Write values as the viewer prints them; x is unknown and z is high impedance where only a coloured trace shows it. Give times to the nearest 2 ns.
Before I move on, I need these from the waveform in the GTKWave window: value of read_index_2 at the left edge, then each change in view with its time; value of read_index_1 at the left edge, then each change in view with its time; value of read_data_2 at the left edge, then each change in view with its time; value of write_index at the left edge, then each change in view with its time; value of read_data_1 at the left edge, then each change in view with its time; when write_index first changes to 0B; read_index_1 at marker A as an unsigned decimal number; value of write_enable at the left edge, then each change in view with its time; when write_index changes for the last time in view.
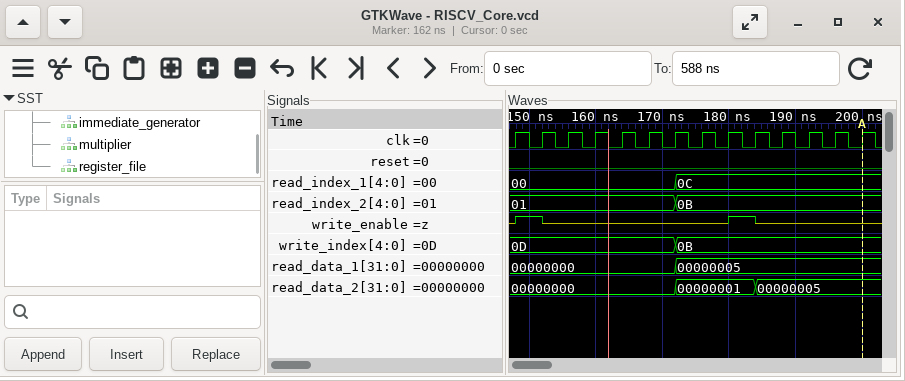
01, 0B at 172 ns
00, 0C at 172 ns
00000000, 00000001 at 172 ns, 00000005 at 184 ns
0D, 0B at 172 ns
00000000, 00000005 at 172 ns
172 ns
12
z, 1 at 148 ns, z at 152 ns, 1 at 180 ns, z at 184 ns
172 ns
